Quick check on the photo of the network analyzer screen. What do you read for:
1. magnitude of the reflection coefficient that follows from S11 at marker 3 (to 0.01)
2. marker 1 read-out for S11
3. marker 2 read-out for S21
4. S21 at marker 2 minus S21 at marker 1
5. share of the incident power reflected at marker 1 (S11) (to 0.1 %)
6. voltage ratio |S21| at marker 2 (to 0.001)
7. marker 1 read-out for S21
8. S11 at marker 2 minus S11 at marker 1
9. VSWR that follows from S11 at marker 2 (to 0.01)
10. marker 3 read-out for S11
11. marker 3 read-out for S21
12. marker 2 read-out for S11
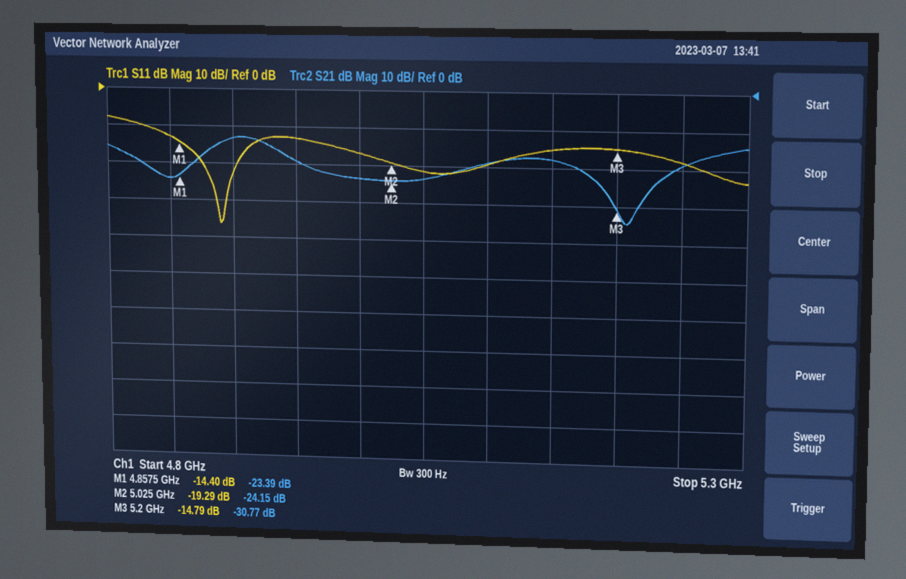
0.18
-14.40 dB
-24.15 dB
-0.76 dB
3.6 %
0.062
-23.39 dB
-4.89 dB
1.24
-14.79 dB
-30.77 dB
-19.29 dB
